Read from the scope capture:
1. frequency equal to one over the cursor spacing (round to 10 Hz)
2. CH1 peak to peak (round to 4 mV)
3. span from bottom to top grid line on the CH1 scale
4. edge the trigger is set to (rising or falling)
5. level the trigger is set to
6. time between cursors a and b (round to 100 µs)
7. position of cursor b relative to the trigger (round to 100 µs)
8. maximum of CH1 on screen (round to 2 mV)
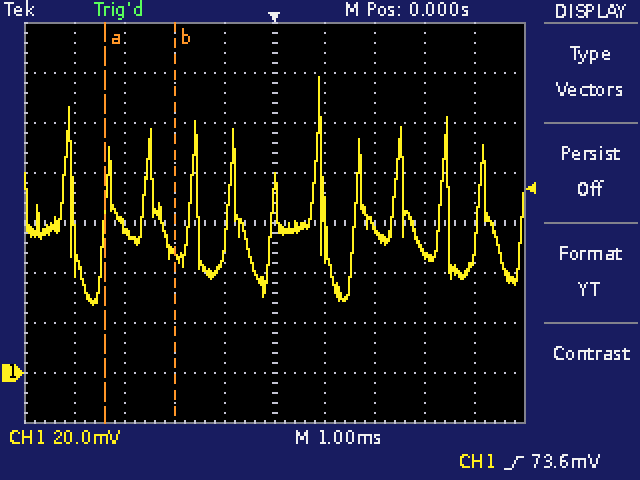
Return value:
710 Hz
92 mV
160 mV
rising
73.6 mV
1.4 ms
-2.0 ms
118 mV
